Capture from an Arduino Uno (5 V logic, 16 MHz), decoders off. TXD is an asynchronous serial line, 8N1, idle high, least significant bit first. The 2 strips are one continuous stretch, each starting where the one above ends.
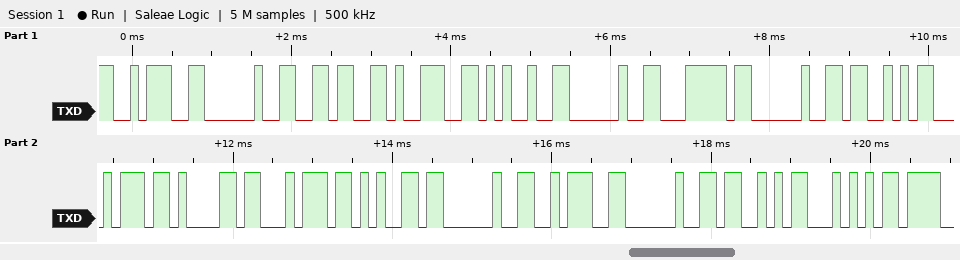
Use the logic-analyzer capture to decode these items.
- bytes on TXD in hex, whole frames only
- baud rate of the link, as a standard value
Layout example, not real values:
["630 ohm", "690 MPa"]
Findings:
["0x3A 0x20 0x36 0x39 0x25 0x20 0x7C 0x20 0x53 0x74 0x61 0x74 0x65 0x20 0x3A 0x20 0x53 0x54", "9600 baud"]
